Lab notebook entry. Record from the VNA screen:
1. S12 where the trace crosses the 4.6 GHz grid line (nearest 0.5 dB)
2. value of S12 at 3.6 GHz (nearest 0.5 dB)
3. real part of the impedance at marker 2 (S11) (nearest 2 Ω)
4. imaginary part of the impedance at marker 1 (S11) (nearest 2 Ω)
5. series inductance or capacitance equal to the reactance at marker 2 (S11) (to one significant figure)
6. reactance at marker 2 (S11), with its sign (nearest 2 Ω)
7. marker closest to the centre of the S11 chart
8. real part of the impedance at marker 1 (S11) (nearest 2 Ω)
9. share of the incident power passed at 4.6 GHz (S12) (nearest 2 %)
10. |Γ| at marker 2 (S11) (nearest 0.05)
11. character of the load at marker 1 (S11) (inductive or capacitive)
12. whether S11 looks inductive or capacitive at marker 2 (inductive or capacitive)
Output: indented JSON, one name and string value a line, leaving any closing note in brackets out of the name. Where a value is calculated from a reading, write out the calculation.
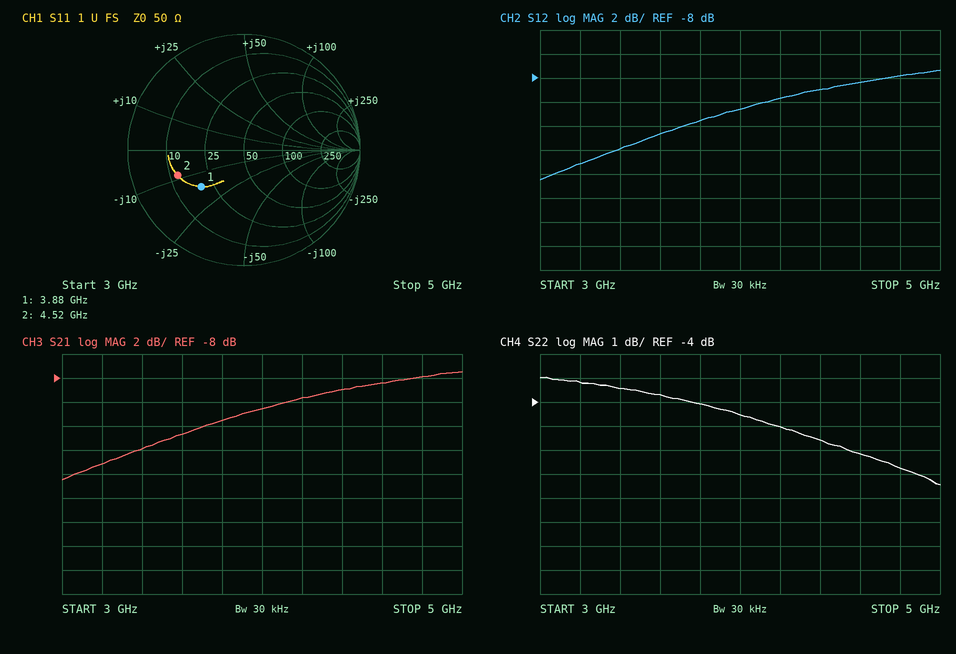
{
  "S12 where the trace crosses the 4.6 GHz grid line": "-8.5 dB",
  "value of S12 at 3.6 GHz": "-12.5 dB",
  "real part of the impedance at marker 2 (S11)": "12 Ω",
  "imaginary part of the impedance at marker 1 (S11)": "-16 Ω",
  "series inductance or capacitance equal to the reactance at marker 2 (S11)": "C = 1/(2π × 4.52 GHz × 8 Ω) ≈ 4 pF",
  "reactance at marker 2 (S11), with its sign": "-8 Ω",
  "marker closest to the centre of the S11 chart": "marker 1",
  "real part of the impedance at marker 1 (S11)": "20 Ω",
  "share of the incident power passed at 4.6 GHz (S12)": "10^(-8.5/10) ≈ 14 %",
  "|Γ| at marker 2 (S11)": "0.60",
  "character of the load at marker 1 (S11)": "capacitive",
  "whether S11 looks inductive or capacitive at marker 2": "capacitive"
}
